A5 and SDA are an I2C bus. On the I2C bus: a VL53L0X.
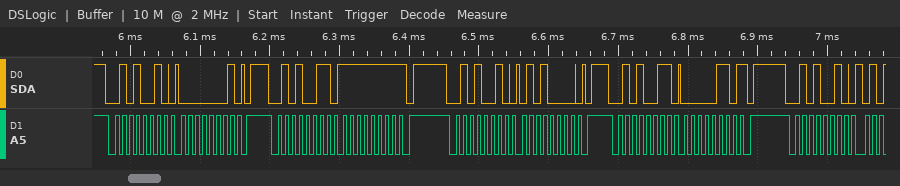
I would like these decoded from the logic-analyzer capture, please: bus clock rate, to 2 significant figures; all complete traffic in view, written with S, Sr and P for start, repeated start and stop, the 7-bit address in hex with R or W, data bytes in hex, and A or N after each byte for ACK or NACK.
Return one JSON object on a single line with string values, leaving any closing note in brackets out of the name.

{"bus clock rate, to 2 significant figures": "100 kHz", "all complete traffic in view, written with S, Sr and P for start, repeated start and stop, the 7-bit address in hex with R or W, data bytes in hex, and A or N after each byte for ACK or NACK": "S 29W A 01 A P S 29R A FF N P S 29W A 50 A P S 29R A 06 N P S 29W A"}
